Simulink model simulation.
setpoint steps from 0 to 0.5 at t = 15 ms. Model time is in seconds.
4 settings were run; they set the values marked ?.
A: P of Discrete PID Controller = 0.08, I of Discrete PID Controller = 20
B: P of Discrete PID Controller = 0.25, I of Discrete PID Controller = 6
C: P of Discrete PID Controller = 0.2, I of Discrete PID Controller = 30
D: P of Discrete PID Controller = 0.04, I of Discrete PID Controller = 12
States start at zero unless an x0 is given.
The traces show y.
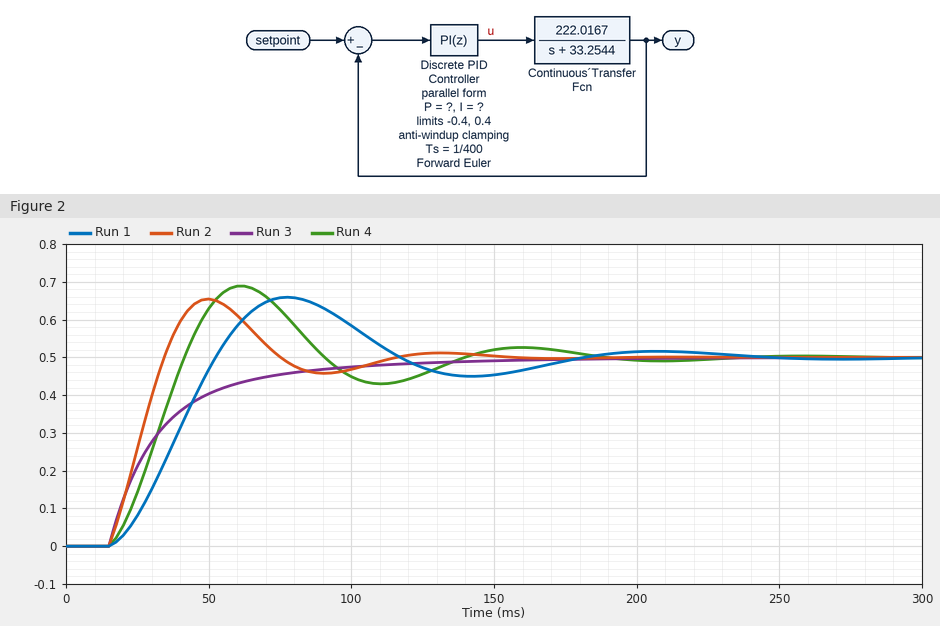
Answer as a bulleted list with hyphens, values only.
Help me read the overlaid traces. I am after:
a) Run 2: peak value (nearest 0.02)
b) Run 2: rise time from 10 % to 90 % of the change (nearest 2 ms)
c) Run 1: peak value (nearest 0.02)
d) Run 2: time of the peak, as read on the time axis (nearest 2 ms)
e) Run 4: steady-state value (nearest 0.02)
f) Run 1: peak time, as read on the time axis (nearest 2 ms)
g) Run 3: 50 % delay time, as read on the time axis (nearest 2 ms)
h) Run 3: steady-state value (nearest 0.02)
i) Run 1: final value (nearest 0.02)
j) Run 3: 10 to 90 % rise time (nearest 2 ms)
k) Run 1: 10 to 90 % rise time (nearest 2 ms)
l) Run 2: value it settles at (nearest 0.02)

- 0.66
- 14 ms
- 0.66
- 50 ms
- 0.50
- 78 ms
- 28 ms
- 0.50
- 0.50
- 54 ms
- 26 ms
- 0.50
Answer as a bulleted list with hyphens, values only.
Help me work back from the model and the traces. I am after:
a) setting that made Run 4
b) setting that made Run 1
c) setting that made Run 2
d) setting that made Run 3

- A
- D
- C
- B
